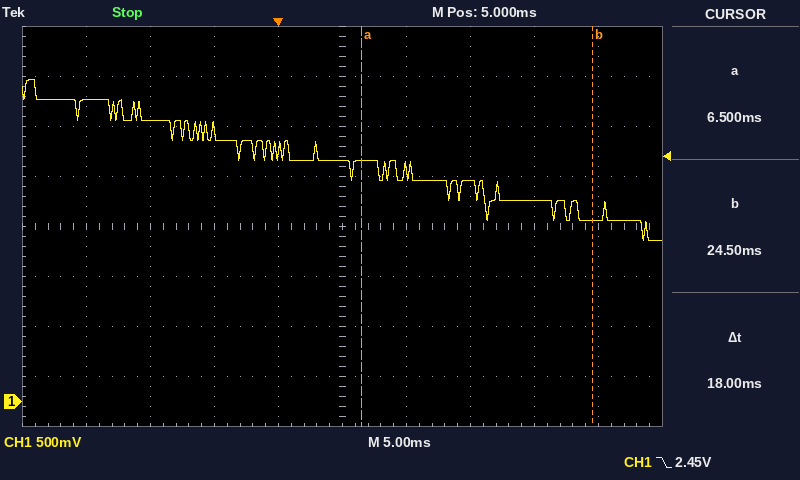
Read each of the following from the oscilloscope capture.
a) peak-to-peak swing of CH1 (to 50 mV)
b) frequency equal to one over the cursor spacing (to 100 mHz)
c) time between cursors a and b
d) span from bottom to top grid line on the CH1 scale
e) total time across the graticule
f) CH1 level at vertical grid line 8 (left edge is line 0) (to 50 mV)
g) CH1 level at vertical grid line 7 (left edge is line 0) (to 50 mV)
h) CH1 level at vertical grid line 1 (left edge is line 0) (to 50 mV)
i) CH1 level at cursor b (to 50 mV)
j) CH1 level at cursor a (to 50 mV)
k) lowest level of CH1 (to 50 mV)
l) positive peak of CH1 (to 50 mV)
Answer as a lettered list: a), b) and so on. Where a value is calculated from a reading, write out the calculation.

a) 3.20 V − (1.60 V) = 1.60 V
b) 1 / 18 ms ≈ 55.6 Hz
c) 18 ms
d) 4 V
e) 50 ms
f) 2.00 V
g) 2.20 V
h) 3.00 V
i) 1.80 V
j) 2.40 V
k) 1.60 V
l) 3.20 V
